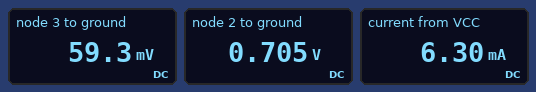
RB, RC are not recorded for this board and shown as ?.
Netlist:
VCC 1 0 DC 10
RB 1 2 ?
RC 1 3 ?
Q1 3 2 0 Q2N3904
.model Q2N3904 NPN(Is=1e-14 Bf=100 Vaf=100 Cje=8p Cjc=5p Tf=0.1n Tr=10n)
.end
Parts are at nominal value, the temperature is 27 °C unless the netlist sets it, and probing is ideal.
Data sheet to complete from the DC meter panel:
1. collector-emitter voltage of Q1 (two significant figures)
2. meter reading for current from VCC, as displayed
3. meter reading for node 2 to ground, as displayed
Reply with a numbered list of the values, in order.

1. 59 mV
2. 6.30 mA
3. 0.705 V
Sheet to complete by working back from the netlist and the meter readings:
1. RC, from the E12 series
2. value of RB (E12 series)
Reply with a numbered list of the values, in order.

1. 1.8 kΩ
2. 12 kΩ
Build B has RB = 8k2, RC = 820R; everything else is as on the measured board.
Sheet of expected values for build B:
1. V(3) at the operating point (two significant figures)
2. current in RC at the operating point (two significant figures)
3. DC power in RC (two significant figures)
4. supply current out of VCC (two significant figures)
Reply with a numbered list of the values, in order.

1. 69 mV
2. 12 mA
3. 120 mW
4. 13 mA
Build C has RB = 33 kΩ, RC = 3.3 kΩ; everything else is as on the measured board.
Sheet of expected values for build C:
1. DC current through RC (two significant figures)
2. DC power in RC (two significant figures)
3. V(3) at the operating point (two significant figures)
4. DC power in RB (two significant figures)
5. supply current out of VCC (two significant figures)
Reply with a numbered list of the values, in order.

1. 3.0 mA
2. 30 mW
3. 69 mV
4. 2.6 mW
5. 3.3 mA
